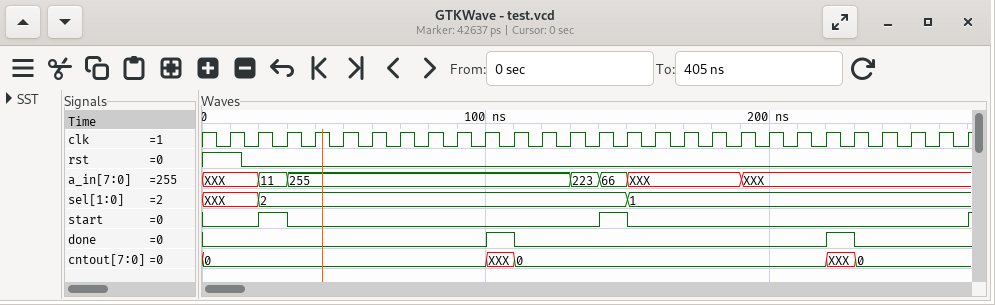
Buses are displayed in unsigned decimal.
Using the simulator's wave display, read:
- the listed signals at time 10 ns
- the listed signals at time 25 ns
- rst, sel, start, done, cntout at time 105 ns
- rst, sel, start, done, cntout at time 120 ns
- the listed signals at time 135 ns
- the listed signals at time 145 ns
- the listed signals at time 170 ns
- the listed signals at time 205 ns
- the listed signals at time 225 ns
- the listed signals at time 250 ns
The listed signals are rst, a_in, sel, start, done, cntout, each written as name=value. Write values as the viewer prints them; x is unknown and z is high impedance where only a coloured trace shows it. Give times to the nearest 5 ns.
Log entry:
rst=1, a_in=XXX, sel=XXX, start=0, done=0, cntout=0
rst=0, a_in=11, sel=2, start=1, done=0, cntout=0
rst=0, sel=2, start=0, done=1, cntout=XXX
rst=0, sel=2, start=0, done=0, cntout=0
rst=0, a_in=223, sel=2, start=0, done=0, cntout=0
rst=0, a_in=66, sel=2, start=1, done=0, cntout=0
rst=0, a_in=XXX, sel=1, start=0, done=0, cntout=0
rst=0, a_in=XXX, sel=1, start=0, done=0, cntout=0
rst=0, a_in=XXX, sel=1, start=0, done=1, cntout=XXX
rst=0, a_in=XXX, sel=1, start=0, done=0, cntout=0
